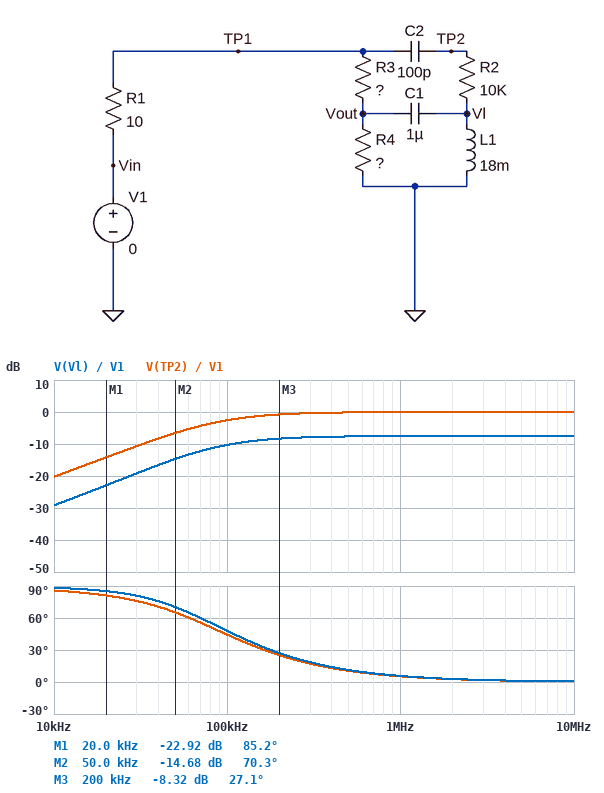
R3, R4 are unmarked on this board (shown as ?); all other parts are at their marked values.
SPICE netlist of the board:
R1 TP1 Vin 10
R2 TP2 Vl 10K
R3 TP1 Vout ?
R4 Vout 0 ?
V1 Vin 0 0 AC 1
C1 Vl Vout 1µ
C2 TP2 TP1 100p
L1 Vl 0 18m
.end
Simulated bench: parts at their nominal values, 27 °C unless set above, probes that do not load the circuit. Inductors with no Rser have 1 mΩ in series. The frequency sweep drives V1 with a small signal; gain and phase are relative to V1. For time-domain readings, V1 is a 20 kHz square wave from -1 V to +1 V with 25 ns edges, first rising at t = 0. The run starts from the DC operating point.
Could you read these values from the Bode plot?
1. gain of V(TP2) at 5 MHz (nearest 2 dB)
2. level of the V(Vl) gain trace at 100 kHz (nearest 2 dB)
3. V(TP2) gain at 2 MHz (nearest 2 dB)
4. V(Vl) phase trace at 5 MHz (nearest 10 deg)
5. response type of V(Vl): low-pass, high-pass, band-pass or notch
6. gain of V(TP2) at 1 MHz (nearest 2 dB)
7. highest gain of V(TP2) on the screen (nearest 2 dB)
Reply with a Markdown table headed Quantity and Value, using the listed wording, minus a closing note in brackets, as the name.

| Quantity | Value |
|---|---|
| gain of V(TP2) at 5 MHz | 0 dB |
| level of the V(Vl) gain trace at 100 kHz | -10 dB |
| V(TP2) gain at 2 MHz | 0 dB |
| V(Vl) phase trace at 5 MHz | 0 deg |
| response type of V(Vl): low-pass, high-pass, band-pass or notch | high-pass |
| gain of V(TP2) at 1 MHz | 0 dB |
| highest gain of V(TP2) on the screen | 0 dB |
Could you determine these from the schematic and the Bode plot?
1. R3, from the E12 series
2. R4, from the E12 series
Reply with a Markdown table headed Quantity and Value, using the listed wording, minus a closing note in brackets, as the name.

| Quantity | Value |
|---|---|
| R3, from the E12 series | 33 kΩ |
| R4, from the E12 series | 5.6 kΩ |
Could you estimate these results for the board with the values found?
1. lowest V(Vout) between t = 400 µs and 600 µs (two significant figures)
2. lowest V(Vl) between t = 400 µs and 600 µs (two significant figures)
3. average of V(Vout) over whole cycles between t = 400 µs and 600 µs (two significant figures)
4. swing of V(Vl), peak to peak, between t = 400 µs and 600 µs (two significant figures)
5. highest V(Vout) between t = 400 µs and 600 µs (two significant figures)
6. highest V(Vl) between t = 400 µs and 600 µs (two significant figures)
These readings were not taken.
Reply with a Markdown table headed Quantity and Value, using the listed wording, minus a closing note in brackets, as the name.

| Quantity | Value |
|---|---|
| lowest V(Vout) between t = 400 µs and 600 µs | -970 mV |
| lowest V(Vl) between t = 400 µs and 600 µs | -840 mV |
| average of V(Vout) over whole cycles between t = 400 µs and 600 µs | -130 mV |
| swing of V(Vl), peak to peak, between t = 400 µs and 600 µs | 1.7 V |
| highest V(Vout) between t = 400 µs and 600 µs | 710 mV |
| highest V(Vl) between t = 400 µs and 600 µs | 840 mV |
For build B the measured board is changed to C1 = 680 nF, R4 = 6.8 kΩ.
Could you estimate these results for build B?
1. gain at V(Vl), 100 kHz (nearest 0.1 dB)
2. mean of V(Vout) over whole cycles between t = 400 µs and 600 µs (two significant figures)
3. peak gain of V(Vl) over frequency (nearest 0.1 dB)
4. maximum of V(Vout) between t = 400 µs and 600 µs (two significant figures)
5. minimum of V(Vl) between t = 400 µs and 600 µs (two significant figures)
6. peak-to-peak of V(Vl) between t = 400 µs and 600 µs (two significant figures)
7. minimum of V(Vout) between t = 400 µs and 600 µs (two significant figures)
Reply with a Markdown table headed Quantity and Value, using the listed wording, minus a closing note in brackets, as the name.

| Quantity | Value |
|---|---|
| gain at V(Vl), 100 kHz | -9.1 dB |
| mean of V(Vout) over whole cycles between t = 400 µs and 600 µs | -150 mV |
| peak gain of V(Vl) over frequency | -6.6 dB |
| maximum of V(Vout) between t = 400 µs and 600 µs | 780 mV |
| minimum of V(Vl) between t = 400 µs and 600 µs | -930 mV |
| peak-to-peak of V(Vl) between t = 400 µs and 600 µs | 1.9 V |
| minimum of V(Vout) between t = 400 µs and 600 µs | -1.1 V |
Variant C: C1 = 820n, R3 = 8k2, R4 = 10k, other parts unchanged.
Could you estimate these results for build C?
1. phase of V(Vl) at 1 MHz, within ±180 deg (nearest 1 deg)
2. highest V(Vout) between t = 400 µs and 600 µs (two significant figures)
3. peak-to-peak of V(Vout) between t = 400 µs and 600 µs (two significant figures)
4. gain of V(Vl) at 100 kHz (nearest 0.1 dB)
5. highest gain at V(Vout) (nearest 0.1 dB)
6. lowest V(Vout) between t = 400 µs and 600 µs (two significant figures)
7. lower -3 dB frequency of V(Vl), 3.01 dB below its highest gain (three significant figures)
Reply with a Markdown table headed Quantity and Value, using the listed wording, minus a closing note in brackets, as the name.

| Quantity | Value |
|---|---|
| phase of V(Vl) at 1 MHz, within ±180 deg | 3 deg |
| highest V(Vout) between t = 400 µs and 600 µs | 900 mV |
| peak-to-peak of V(Vout) between t = 400 µs and 600 µs | 2.8 V |
| gain of V(Vl) at 100 kHz | -4.2 dB |
| highest gain at V(Vout) | -3.2 dB |
| lowest V(Vout) between t = 400 µs and 600 µs | -1.9 V |
| lower -3 dB frequency of V(Vl), 3.01 dB below its highest gain | 49.8 kHz |
